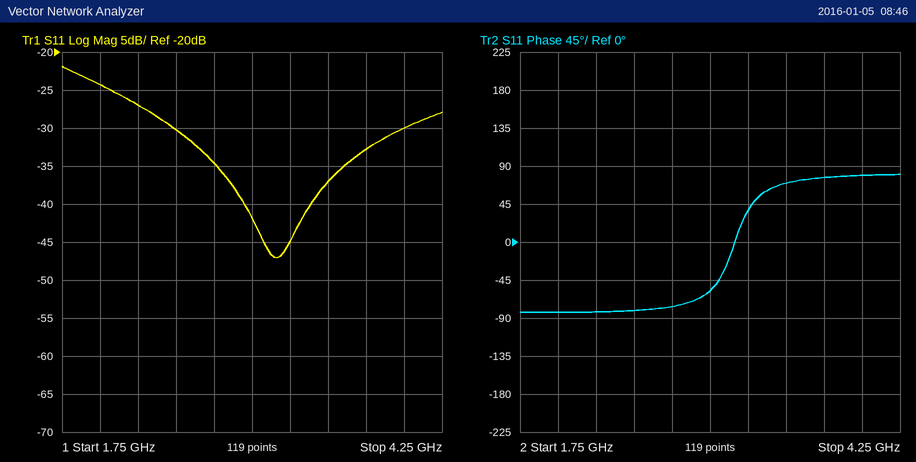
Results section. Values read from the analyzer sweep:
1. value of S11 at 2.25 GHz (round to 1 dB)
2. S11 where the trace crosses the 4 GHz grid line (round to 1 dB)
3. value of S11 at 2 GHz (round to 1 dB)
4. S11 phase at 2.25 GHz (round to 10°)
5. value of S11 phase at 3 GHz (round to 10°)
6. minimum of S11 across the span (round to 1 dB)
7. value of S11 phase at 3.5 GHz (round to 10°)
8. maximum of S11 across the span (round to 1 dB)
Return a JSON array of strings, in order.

["-27 dB", "-30 dB", "-24 dB", "-80°", "-60°", "-47 dB", "70°", "-22 dB"]
